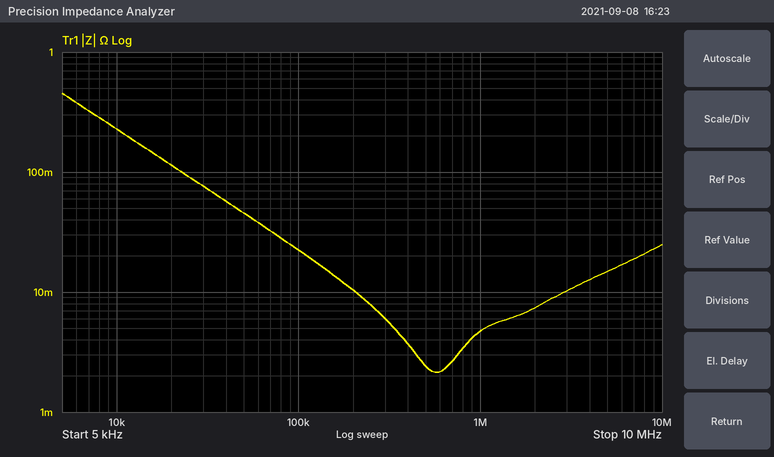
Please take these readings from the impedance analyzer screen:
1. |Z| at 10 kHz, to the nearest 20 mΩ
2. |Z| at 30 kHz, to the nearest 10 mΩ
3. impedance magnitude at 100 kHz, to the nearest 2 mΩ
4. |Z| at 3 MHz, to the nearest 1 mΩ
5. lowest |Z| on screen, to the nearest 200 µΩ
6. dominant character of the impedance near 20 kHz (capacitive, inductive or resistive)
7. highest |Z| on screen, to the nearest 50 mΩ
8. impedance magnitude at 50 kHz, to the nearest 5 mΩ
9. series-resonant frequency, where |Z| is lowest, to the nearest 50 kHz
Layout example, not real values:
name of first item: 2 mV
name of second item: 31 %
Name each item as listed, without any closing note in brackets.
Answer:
|Z| at 10 kHz, to the nearest 20 mΩ: 220 mΩ
|Z| at 30 kHz, to the nearest 10 mΩ: 80 mΩ
impedance magnitude at 100 kHz, to the nearest 2 mΩ: 22 mΩ
|Z| at 3 MHz, to the nearest 1 mΩ: 10 mΩ
lowest |Z| on screen, to the nearest 200 µΩ: 2.2 mΩ
dominant character of the impedance near 20 kHz: capacitive
highest |Z| on screen, to the nearest 50 mΩ: 450 mΩ
impedance magnitude at 50 kHz, to the nearest 5 mΩ: 45 mΩ
series-resonant frequency, where |Z| is lowest, to the nearest 50 kHz: 550 kHz
